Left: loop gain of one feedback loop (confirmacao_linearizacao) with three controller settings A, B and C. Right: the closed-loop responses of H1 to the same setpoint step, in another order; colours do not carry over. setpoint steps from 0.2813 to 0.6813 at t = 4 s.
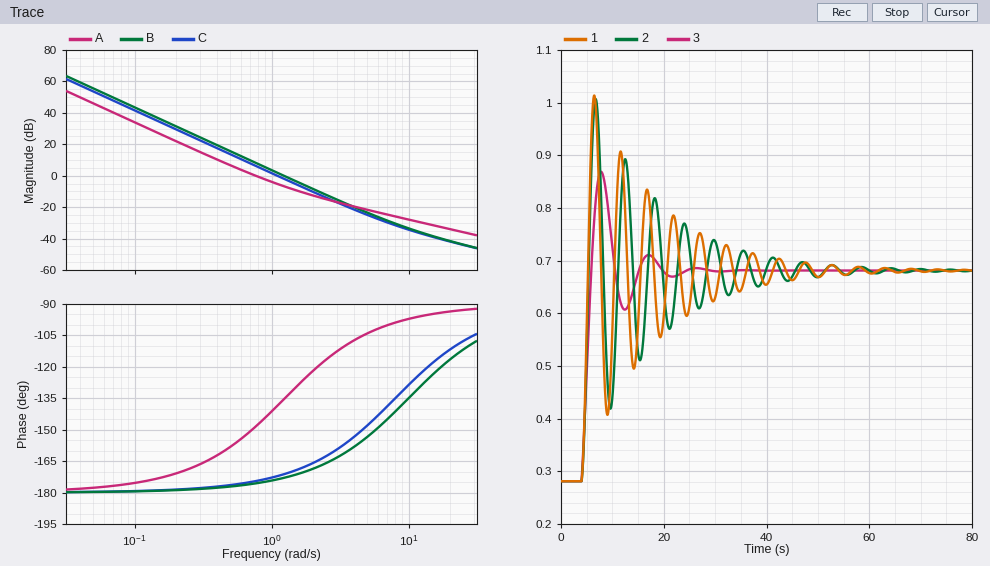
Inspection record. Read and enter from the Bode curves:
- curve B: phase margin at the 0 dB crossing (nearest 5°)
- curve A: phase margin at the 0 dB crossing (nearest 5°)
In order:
5°
30°
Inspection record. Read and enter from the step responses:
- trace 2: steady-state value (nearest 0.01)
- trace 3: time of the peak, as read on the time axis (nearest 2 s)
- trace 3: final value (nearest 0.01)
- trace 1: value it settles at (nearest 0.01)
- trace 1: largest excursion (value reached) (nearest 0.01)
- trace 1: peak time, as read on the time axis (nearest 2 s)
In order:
0.68
8 s
0.68
0.68
1.01
6 s
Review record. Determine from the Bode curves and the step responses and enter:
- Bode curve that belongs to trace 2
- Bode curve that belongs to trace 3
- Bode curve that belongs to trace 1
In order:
C
A
B
